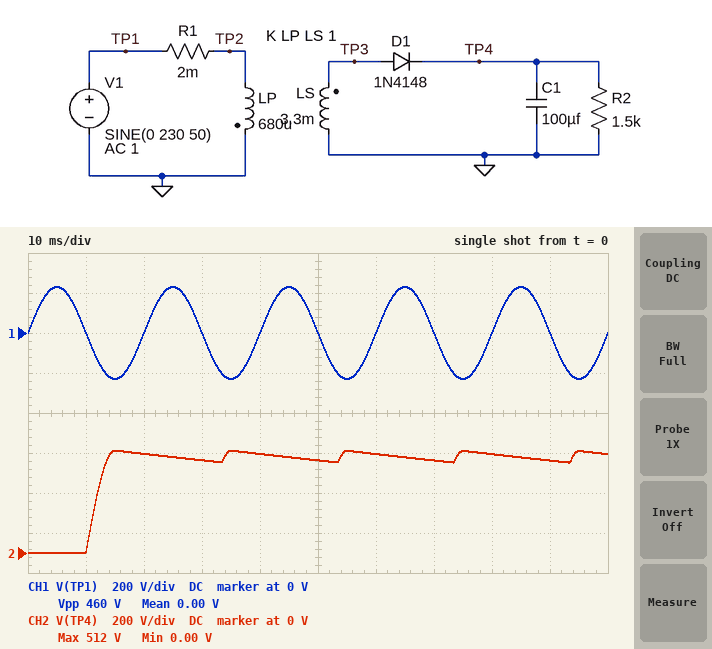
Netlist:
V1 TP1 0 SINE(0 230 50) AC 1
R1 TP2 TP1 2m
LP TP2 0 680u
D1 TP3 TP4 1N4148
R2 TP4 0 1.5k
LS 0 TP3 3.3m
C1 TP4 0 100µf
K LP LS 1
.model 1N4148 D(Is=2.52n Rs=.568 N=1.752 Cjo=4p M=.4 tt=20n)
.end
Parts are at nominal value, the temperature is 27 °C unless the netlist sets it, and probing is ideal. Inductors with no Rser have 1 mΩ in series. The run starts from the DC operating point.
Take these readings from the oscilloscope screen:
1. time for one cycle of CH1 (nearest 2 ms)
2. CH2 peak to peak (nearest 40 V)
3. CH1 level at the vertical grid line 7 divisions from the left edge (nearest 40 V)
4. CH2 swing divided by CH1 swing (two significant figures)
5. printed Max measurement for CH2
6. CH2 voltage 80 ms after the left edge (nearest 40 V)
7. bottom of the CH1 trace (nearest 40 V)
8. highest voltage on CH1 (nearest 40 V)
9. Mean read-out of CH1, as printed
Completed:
20 ms
520 V
0 V
1.1
512 V
480 V
-240 V
240 V
0.00 V
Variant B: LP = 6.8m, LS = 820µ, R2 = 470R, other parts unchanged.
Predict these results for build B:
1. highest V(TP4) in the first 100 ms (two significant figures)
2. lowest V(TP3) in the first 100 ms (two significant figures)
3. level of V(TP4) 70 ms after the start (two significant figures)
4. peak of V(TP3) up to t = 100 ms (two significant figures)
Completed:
79 V
-80 V
58 V
80 V
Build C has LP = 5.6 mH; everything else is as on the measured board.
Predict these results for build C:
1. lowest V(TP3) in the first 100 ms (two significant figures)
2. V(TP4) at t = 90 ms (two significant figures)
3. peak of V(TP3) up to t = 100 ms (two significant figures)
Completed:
-180 V
160 V
180 V
